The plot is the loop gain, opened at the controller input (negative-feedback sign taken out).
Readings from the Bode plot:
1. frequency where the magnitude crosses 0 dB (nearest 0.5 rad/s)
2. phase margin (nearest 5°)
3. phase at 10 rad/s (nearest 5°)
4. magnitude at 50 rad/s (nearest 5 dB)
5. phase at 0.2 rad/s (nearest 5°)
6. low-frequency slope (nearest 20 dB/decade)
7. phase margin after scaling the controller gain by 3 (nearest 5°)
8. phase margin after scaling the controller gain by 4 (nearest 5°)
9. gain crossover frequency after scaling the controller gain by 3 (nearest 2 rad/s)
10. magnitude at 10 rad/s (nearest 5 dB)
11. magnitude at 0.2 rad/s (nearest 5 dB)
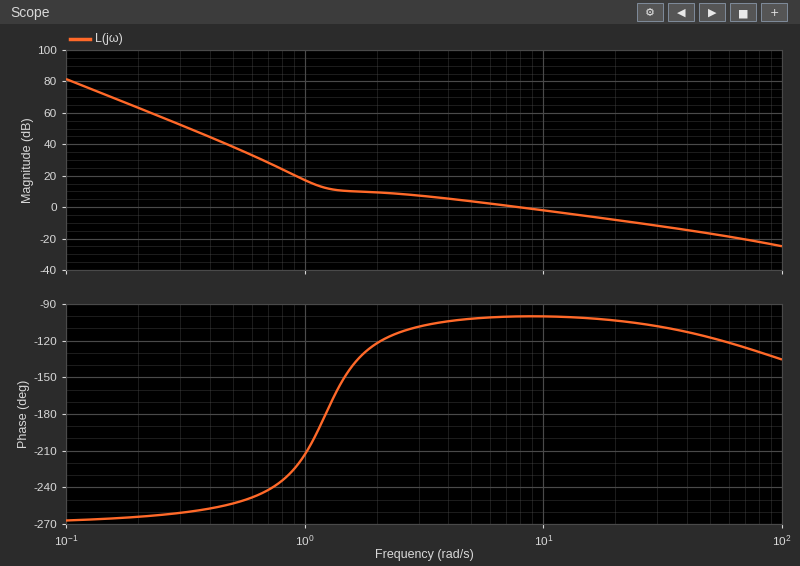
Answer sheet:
8.0 rad/s
80°
-100°
-15 dB
-265°
-60 dB/decade
75°
70°
24 rad/s
0 dB
65 dB
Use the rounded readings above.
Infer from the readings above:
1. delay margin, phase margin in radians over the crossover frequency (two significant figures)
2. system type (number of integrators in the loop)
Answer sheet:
0.17 s
3
